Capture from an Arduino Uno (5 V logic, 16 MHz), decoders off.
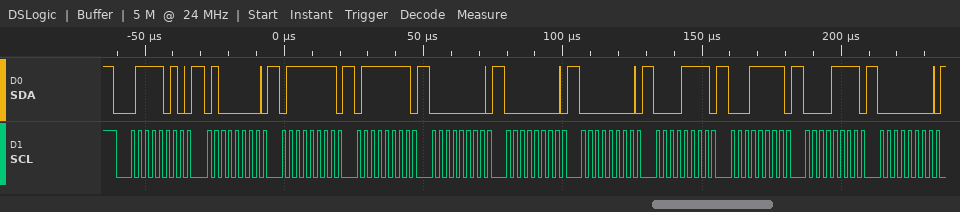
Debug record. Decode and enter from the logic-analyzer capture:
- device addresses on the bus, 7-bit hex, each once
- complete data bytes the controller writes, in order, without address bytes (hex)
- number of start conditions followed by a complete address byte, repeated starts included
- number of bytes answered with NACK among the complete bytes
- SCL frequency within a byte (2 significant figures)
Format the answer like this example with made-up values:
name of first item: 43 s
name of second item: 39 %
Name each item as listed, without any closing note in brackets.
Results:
device addresses on the bus, 7-bit hex, each once: 0x3D
complete data bytes the controller writes, in order, without address bytes: 40 7F 7F 00 00 00 0F 1F 0F 00
number of start conditions followed by a complete address byte, repeated starts included: 1
number of bytes answered with NACK among the complete bytes: 0
SCL frequency within a byte: 400 kHz
